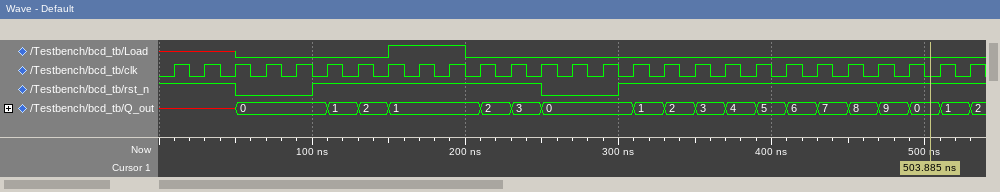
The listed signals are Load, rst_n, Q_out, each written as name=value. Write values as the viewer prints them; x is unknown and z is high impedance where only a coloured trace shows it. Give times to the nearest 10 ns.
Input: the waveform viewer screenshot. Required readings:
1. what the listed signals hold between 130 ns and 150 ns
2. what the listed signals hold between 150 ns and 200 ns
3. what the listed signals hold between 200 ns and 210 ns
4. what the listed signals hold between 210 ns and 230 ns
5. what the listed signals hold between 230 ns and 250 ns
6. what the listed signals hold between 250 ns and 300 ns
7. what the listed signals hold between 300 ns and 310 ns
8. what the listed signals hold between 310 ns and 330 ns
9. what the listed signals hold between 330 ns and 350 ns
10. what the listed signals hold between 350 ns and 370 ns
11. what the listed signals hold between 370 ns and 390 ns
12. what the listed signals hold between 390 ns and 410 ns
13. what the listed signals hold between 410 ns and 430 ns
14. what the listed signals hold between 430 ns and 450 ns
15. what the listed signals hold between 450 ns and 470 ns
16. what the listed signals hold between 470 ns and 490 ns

Load=0, rst_n=1, Q_out=2
Load=1, rst_n=1, Q_out=1
Load=0, rst_n=1, Q_out=1
Load=0, rst_n=1, Q_out=2
Load=0, rst_n=1, Q_out=3
Load=0, rst_n=0, Q_out=0
Load=0, rst_n=1, Q_out=0
Load=0, rst_n=1, Q_out=1
Load=0, rst_n=1, Q_out=2
Load=0, rst_n=1, Q_out=3
Load=0, rst_n=1, Q_out=4
Load=0, rst_n=1, Q_out=5
Load=0, rst_n=1, Q_out=6
Load=0, rst_n=1, Q_out=7
Load=0, rst_n=1, Q_out=8
Load=0, rst_n=1, Q_out=9
